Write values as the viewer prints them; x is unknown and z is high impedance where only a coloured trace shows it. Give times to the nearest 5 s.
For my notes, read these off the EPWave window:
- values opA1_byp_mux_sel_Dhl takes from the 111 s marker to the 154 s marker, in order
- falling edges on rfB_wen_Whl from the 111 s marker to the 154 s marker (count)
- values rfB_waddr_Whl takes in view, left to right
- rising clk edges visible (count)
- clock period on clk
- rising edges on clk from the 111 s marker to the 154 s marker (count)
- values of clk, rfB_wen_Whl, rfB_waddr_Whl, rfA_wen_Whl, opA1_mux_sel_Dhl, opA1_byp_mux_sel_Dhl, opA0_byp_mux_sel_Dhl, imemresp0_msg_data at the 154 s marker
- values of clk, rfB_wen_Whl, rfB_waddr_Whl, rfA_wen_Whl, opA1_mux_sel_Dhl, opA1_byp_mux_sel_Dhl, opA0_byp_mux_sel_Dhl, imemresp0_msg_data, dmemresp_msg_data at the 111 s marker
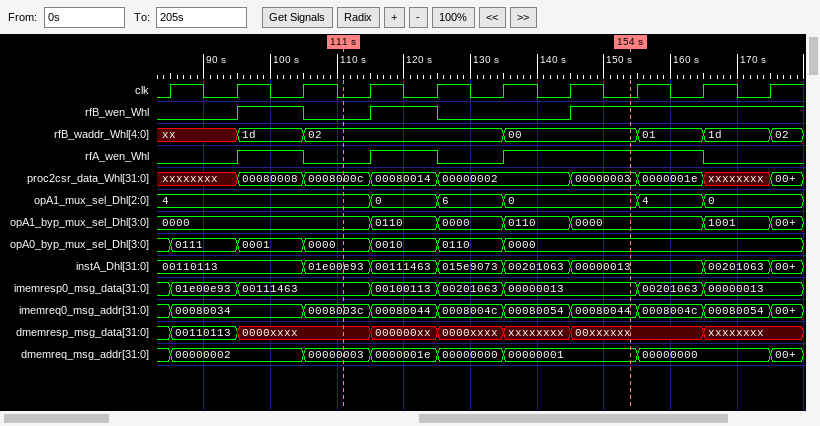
0000, 0110, 0000, 0110, 0000
1
xx, 1d, 02, 00, 01, 1d, 02
10
10 s
4
clk=0, rfB_wen_Whl=1, rfB_waddr_Whl=00, rfA_wen_Whl=1, opA1_mux_sel_Dhl=0, opA1_byp_mux_sel_Dhl=0000, opA0_byp_mux_sel_Dhl=0000, imemresp0_msg_data=00000013
clk=0, rfB_wen_Whl=0, rfB_waddr_Whl=02, rfA_wen_Whl=0, opA1_mux_sel_Dhl=4, opA1_byp_mux_sel_Dhl=0000, opA0_byp_mux_sel_Dhl=0000, imemresp0_msg_data=00111463, dmemresp_msg_data=0000xxxx
